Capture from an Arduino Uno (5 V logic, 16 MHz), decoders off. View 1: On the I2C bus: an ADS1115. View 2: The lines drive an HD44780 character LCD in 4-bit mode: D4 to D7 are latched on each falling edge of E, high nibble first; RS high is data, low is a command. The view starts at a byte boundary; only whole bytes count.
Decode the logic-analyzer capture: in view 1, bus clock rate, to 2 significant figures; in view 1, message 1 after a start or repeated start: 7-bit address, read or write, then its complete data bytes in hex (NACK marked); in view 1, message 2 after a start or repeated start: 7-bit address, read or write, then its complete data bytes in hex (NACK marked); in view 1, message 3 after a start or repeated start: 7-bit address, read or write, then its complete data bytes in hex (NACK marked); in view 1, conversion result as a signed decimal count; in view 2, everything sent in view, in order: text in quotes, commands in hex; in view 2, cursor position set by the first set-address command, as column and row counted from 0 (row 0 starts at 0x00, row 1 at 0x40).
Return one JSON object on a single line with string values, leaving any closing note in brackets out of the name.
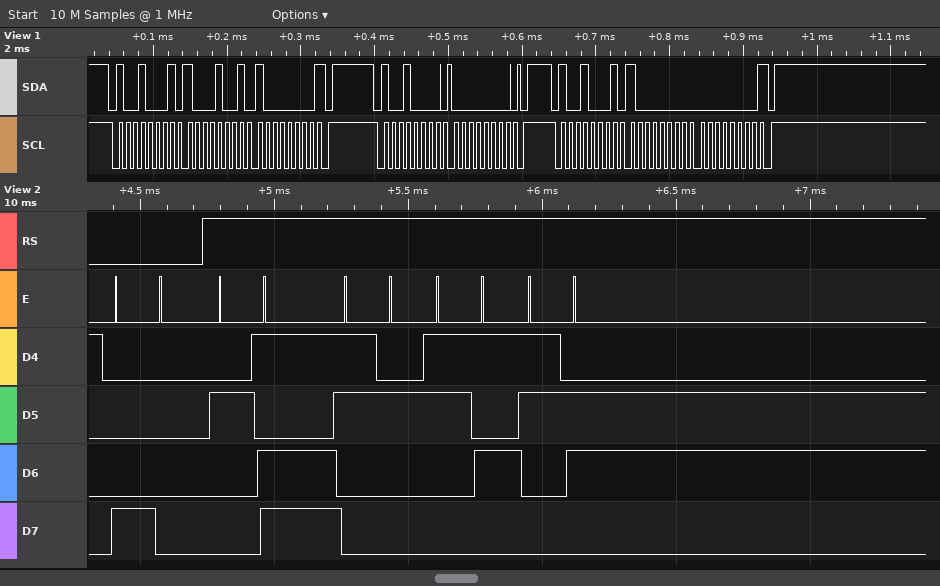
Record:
{"in view 1, bus clock rate, to 2 significant figures": "100 kHz", "in view 1, message 1 after a start or repeated start: 7-bit address, read or write, then its complete data bytes in hex": "0x48 read: 89 80 NACK", "in view 1, message 2 after a start or repeated start: 7-bit address, read or write, then its complete data bytes in hex": "0x48 write: 00", "in view 1, message 3 after a start or repeated start: 7-bit address, read or write, then its complete data bytes in hex": "0x48 read: 80 00 NACK", "in view 1, conversion result as a signed decimal count": "-32768", "in view 2, everything sent in view, in order: text in quotes, commands in hex": "0x80 \"-256\"", "in view 2, cursor position set by the first set-address command, as column and row counted from 0": "column 0, row 0"}
